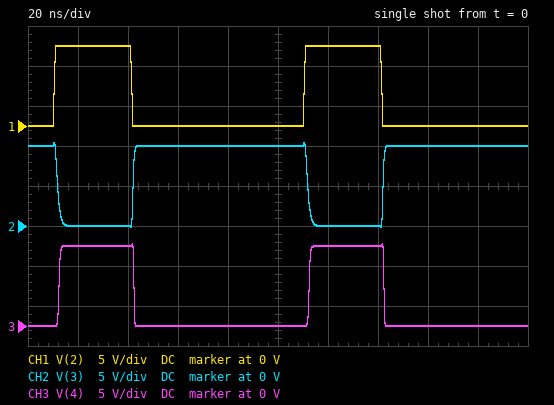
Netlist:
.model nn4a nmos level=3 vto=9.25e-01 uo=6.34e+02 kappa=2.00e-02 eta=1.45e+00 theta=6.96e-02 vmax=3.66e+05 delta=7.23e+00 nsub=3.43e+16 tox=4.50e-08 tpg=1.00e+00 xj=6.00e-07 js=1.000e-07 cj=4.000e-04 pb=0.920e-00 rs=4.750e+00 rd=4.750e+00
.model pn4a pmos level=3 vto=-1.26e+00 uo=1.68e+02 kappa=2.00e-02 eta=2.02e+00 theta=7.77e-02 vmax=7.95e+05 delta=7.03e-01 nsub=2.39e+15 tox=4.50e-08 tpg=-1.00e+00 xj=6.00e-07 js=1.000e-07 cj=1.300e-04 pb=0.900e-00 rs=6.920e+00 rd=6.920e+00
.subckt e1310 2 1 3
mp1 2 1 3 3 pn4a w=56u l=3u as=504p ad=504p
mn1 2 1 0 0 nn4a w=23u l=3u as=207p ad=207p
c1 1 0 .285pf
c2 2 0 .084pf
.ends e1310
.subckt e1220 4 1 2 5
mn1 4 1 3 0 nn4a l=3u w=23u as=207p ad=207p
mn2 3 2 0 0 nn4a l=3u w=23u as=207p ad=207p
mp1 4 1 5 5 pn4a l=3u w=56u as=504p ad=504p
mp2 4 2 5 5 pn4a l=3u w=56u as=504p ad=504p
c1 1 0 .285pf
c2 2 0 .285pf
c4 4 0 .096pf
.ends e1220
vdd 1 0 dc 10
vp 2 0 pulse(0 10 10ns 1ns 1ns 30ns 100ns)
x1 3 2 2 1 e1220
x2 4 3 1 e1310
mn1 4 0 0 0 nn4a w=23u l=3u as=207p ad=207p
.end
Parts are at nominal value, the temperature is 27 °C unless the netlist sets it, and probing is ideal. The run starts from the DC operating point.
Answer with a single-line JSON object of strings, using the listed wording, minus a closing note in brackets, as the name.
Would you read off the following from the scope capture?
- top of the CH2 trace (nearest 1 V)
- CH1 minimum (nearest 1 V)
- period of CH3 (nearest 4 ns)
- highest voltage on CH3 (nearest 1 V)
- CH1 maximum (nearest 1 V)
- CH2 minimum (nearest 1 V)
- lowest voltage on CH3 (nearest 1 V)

{"top of the CH2 trace": "10 V", "CH1 minimum": "0 V", "period of CH3": "100 ns", "highest voltage on CH3": "10 V", "CH1 maximum": "10 V", "CH2 minimum": "0 V", "lowest voltage on CH3": "0 V"}
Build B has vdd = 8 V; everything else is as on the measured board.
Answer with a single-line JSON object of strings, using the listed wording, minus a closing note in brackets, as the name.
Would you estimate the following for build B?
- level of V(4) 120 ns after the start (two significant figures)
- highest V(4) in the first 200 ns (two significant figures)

{"level of V(4) 120 ns after the start": "8.0 V", "highest V(4) in the first 200 ns": "8.3 V"}
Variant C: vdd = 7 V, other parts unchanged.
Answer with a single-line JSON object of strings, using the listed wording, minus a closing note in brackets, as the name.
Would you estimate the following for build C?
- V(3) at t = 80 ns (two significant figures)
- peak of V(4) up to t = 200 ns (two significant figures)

{"V(3) at t = 80 ns": "7.0 V", "peak of V(4) up to t = 200 ns": "7.3 V"}
